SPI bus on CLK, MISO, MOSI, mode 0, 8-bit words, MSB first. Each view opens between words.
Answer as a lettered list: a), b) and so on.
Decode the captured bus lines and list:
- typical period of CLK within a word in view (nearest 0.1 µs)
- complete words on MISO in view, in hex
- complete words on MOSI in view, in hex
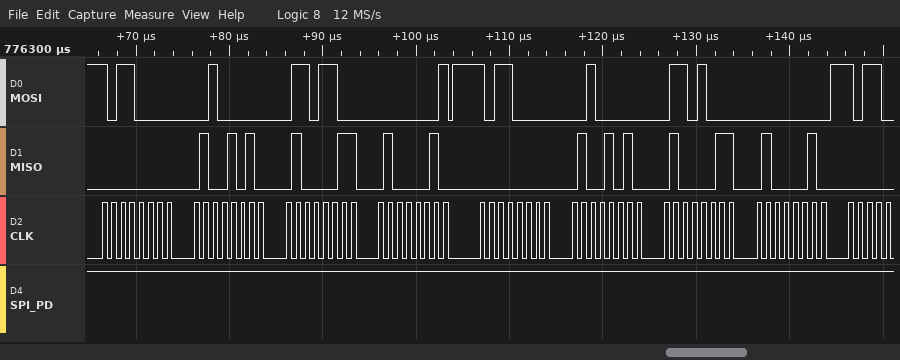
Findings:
a) 1 µs
b) 00, 4A, 43, 42, 00, 4A, 43, 42
c) B0, 20, 6C, 01, B0, 20, 68, 00
